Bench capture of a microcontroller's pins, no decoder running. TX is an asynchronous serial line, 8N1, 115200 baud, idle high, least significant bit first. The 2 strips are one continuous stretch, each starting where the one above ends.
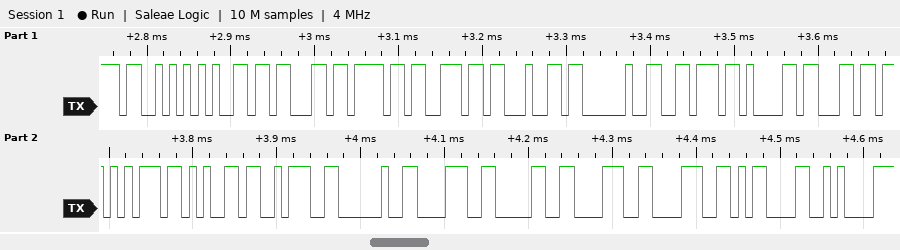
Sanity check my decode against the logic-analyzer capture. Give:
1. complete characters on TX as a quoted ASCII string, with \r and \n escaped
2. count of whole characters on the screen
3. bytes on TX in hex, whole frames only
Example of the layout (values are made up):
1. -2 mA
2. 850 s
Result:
1. "Second value: 8088\r\n"
2. 20
3. 0x53 0x65 0x63 0x6F 0x6E 0x64 0x20 0x76 0x61 0x6C 0x75 0x65 0x3A 0x20 0x38 0x30 0x38 0x38 0x0D 0x0A
